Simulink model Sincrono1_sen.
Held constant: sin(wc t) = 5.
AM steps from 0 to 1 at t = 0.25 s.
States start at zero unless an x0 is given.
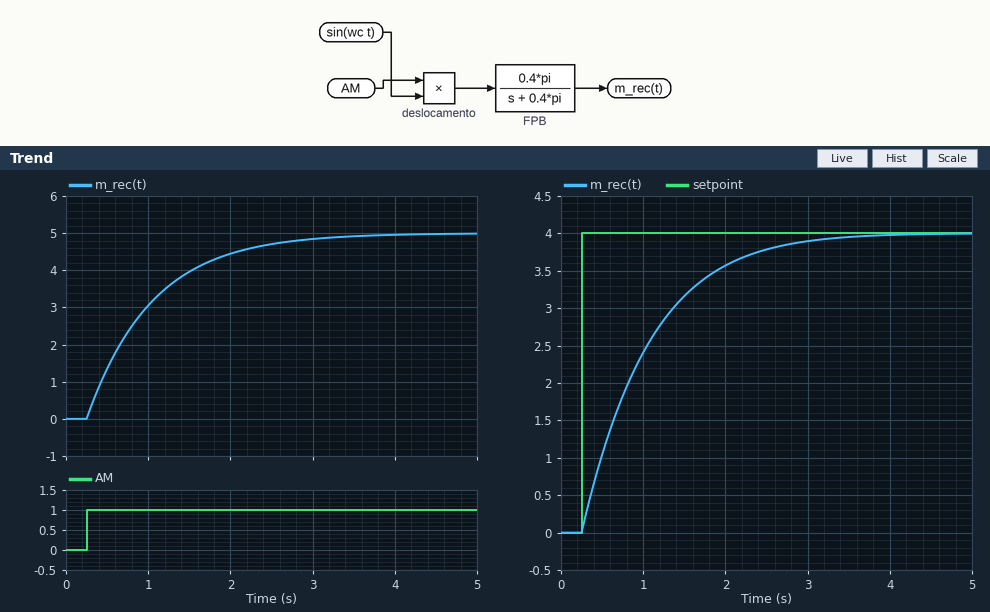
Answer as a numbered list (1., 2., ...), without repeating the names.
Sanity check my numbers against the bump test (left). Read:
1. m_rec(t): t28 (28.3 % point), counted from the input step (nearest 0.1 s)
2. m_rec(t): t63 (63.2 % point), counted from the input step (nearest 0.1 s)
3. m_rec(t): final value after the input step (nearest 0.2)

1. 0.3 s
2. 0.8 s
3. 5.0
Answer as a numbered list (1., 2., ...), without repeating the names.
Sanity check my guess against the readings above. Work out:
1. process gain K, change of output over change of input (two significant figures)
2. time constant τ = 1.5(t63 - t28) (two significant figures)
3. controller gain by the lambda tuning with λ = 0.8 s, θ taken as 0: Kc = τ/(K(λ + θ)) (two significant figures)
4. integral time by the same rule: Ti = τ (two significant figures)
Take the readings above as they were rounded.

1. 5.0
2. 0.75 s
3. 0.19
4. 0.75 s
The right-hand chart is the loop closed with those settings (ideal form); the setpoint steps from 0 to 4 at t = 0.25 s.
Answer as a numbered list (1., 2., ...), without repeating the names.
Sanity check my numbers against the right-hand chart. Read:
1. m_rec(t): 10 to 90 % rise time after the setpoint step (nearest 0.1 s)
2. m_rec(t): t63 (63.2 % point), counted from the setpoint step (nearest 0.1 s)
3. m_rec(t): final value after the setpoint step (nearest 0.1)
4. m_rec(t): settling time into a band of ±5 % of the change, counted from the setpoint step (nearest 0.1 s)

1. 1.7 s
2. 0.8 s
3. 4.0
4. 2.3 s
